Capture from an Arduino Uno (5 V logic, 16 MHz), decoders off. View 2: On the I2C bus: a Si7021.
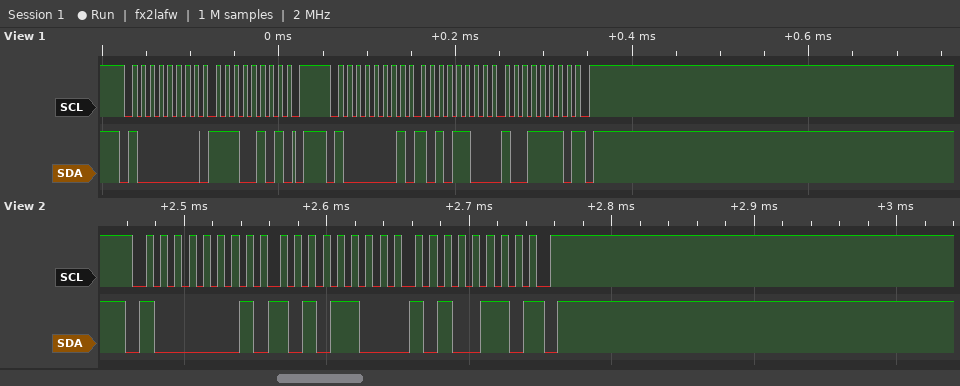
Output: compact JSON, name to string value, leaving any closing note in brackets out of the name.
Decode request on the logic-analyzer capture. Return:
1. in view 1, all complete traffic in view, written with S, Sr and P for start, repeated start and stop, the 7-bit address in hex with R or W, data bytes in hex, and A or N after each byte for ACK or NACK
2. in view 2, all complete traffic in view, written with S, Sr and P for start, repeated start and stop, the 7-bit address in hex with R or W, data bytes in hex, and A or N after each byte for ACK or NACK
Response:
{"in view 1, all complete traffic in view, written with S, Sr and P for start, repeated start and stop, the 7-bit address in hex with R or W, data bytes in hex, and A or N after each byte for ACK or NACK": "S 40W A E5 A P S 40R A AC A 9E N P", "in view 2, all complete traffic in view, written with S, Sr and P for start, repeated start and stop, the 7-bit address in hex with R or W, data bytes in hex, and A or N after each byte for ACK or NACK": "S 40R A AC A A6 N P"}
